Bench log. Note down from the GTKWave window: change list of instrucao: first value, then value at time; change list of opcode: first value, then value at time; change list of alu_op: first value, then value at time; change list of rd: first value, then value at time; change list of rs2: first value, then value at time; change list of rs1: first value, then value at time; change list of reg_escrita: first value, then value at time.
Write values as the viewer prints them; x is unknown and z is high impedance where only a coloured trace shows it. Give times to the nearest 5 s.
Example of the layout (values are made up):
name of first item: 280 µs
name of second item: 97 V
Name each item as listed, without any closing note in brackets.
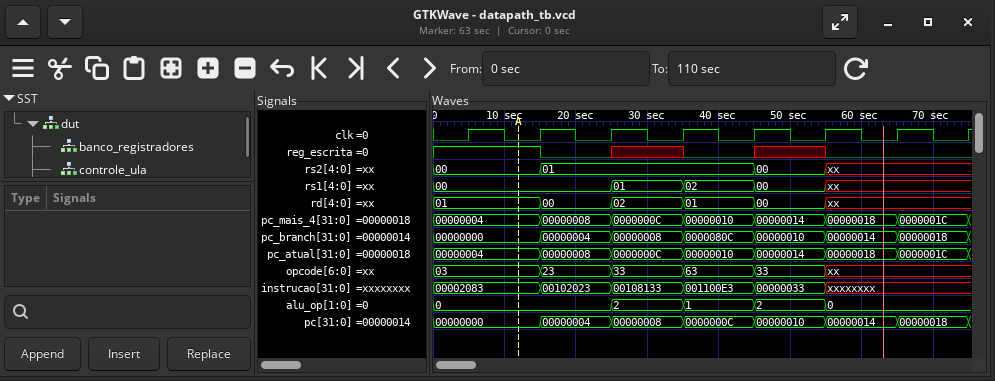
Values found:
change list of instrucao: first value, then value at time: 00002083, 00102023 at 15 s, 00108133 at 25 s, 001100E3 at 35 s, 00000033 at 45 s, xxxxxxxx at 55 s
change list of opcode: first value, then value at time: 03, 23 at 15 s, 33 at 25 s, 63 at 35 s, 33 at 45 s, xx at 55 s
change list of alu_op: first value, then value at time: 0, 2 at 25 s, 1 at 35 s, 2 at 45 s, 0 at 55 s
change list of rd: first value, then value at time: 01, 00 at 15 s, 02 at 25 s, 01 at 35 s, 00 at 45 s, xx at 55 s
change list of rs2: first value, then value at time: 00, 01 at 15 s, 00 at 45 s, xx at 55 s
change list of rs1: first value, then value at time: 00, 01 at 25 s, 02 at 35 s, 00 at 45 s, xx at 55 s
change list of reg_escrita: first value, then value at time: 1, 0 at 15 s, x at 25 s, 0 at 35 s, x at 45 s, 0 at 55 s
